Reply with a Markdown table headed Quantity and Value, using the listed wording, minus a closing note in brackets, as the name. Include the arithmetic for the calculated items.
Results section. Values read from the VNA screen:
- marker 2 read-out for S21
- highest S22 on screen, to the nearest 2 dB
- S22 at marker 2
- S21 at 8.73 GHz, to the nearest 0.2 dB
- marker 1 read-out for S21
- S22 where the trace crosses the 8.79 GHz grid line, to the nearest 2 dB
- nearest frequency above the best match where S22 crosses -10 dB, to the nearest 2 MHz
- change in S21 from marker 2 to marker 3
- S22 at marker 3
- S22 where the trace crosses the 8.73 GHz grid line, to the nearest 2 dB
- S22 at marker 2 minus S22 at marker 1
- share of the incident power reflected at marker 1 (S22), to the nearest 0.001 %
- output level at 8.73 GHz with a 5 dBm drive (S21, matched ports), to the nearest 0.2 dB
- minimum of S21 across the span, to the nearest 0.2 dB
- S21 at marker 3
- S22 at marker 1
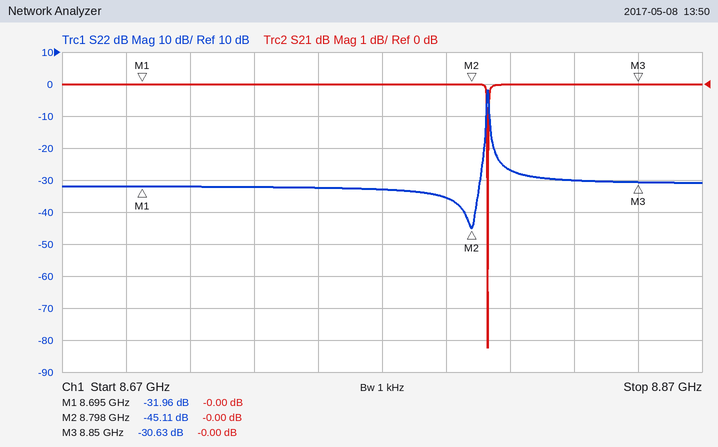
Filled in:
| Quantity | Value |
|---|---|
| marker 2 read-out for S21 | -0.00 dB |
| highest S22 on screen, to the nearest 2 dB | -2 dB |
| S22 at marker 2 | -45.11 dB |
| S21 at 8.73 GHz, to the nearest 0.2 dB | 0.0 dB |
| marker 1 read-out for S21 | -0.00 dB |
| S22 where the trace crosses the 8.79 GHz grid line, to the nearest 2 dB | -36 dB |
| nearest frequency above the best match where S22 crosses -10 dB, to the nearest 2 MHz | 8.802 GHz |
| change in S21 from marker 2 to marker 3 | -0 − (-0) = 0.00 dB |
| S22 at marker 3 | -30.63 dB |
| S22 where the trace crosses the 8.73 GHz grid line, to the nearest 2 dB | -32 dB |
| S22 at marker 2 minus S22 at marker 1 | -45.11 − (-31.96) = -13.15 dB |
| share of the incident power reflected at marker 1 (S22), to the nearest 0.001 % | 10^(-31.96/10) ≈ 0.064 % |
| output level at 8.73 GHz with a 5 dBm drive (S21, matched ports), to the nearest 0.2 dB | 5 dBm + (0.0 dB) = 5.0 dBm |
| minimum of S21 across the span, to the nearest 0.2 dB | -8.2 dB |
| S21 at marker 3 | -0.00 dB |
| S22 at marker 1 | -31.96 dB |
